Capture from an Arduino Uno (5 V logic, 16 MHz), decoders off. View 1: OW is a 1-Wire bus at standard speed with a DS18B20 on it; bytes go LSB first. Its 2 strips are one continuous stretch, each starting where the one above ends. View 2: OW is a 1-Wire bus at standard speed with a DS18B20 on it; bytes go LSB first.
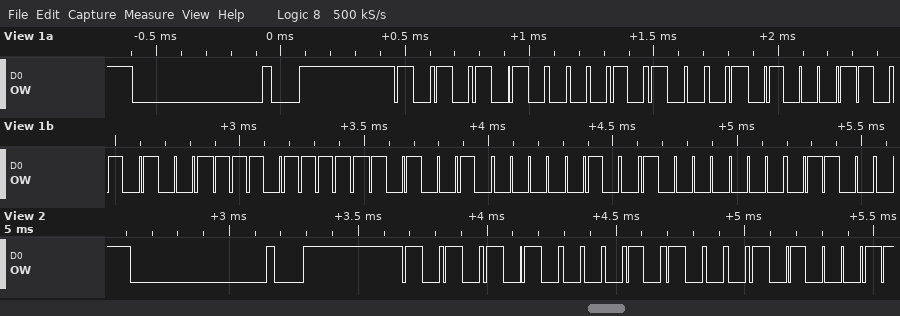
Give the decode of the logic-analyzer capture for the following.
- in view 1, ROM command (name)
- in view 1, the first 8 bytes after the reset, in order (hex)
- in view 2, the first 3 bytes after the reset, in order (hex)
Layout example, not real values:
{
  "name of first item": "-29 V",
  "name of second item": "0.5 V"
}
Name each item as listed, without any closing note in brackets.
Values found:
{
  "in view 1, ROM command": "Match ROM",
  "in view 1, the first 8 bytes after the reset, in order": "55 28 8A 95 F7 4B 20 01",
  "in view 2, the first 3 bytes after the reset, in order": "55 28 8A"
}
